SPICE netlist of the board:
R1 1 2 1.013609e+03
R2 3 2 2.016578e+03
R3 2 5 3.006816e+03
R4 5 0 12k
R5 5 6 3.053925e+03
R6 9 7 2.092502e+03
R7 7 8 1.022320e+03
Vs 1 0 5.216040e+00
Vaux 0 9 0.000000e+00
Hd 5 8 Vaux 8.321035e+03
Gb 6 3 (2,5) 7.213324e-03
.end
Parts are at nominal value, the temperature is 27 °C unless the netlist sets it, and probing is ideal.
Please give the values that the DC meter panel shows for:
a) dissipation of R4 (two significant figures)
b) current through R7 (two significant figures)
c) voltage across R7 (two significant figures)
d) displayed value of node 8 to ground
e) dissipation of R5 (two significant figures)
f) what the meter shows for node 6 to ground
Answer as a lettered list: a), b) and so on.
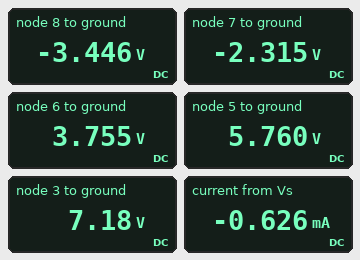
a) 2.8 mW
b) 1.1 mA
c) 1.1 V
d) -3.446 V
e) 1.3 mW
f) 3.755 V
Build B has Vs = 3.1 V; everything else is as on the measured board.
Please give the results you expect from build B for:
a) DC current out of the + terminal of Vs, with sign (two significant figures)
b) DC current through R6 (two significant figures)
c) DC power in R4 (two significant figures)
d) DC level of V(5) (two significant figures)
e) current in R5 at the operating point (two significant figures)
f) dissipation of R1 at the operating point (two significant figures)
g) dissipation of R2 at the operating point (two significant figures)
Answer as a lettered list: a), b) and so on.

a) -370 µA
b) 660 µA
c) 980 µW
d) 3.4 V
e) 390 µA
f) 140 µW
g) 310 µW
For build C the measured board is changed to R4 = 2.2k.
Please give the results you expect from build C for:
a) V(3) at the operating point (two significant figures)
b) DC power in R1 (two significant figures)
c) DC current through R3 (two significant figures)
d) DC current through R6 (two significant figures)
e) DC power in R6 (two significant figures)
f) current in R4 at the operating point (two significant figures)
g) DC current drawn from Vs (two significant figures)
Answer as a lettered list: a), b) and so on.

a) 1.7 V
b) 1.3 mW
c) 54 µA
d) 820 µA
e) 1.4 mW
f) 1.9 mA
g) 1.1 mA
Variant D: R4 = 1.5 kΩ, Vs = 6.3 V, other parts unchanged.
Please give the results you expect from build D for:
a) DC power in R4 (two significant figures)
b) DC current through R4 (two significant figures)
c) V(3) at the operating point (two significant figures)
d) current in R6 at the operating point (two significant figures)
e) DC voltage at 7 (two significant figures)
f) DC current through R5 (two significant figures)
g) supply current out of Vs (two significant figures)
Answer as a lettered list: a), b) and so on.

a) 13 mW
b) 3.0 mA
c) -320 mV
d) 860 µA
e) -1.8 V
f) 2.2 mA
g) 2.1 mA
